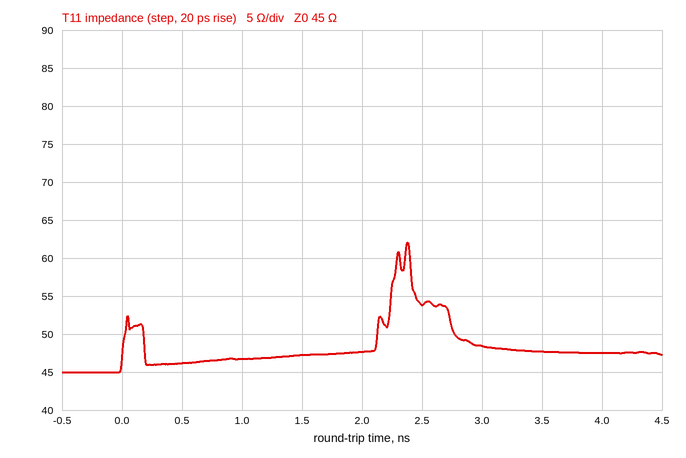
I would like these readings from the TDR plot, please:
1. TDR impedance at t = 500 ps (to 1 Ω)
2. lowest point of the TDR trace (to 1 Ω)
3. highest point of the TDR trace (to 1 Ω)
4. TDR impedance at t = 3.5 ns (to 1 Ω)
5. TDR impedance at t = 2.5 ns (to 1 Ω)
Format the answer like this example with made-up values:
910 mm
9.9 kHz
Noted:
46 Ω
45 Ω
62 Ω
48 Ω
54 Ω
